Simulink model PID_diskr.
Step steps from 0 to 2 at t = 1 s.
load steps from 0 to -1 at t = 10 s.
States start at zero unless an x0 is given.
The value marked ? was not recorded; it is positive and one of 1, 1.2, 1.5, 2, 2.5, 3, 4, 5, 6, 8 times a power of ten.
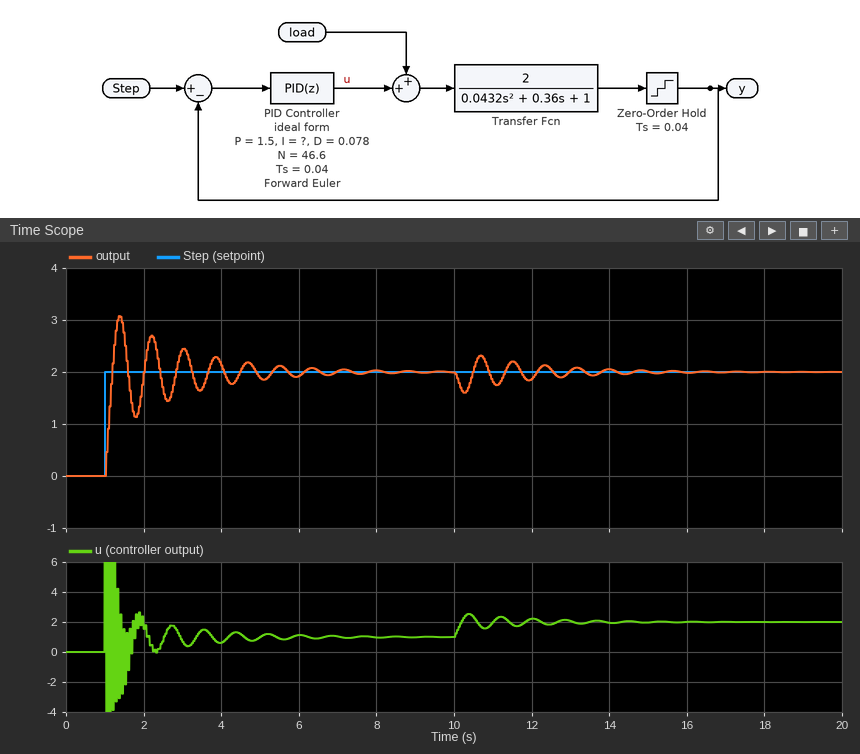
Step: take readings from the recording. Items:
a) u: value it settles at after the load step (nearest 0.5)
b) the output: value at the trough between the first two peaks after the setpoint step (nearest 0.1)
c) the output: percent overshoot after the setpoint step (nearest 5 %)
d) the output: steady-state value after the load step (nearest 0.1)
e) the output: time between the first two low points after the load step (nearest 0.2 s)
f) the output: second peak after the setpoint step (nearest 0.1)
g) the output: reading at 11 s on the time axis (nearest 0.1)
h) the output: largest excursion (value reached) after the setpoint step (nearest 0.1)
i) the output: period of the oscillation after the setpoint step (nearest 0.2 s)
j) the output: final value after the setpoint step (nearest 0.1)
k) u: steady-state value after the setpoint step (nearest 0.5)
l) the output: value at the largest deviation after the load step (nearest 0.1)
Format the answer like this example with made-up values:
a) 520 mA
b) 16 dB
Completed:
a) 2.0
b) 1.1
c) 55 %
d) 2.0
e) 0.8 s
f) 2.7
g) 1.8
h) 3.1
i) 0.8 s
j) 2.0
k) 1.0
l) 1.6
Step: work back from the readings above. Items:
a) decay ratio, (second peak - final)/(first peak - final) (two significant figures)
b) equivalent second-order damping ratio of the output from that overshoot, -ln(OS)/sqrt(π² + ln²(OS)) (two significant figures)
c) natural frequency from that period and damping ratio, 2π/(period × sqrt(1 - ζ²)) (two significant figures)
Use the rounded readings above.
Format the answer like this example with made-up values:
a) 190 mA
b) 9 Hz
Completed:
a) 0.64
b) 0.19
c) 8.0 rad/s
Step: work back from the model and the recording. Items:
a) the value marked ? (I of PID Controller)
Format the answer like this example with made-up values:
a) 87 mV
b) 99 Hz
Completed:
a) 10
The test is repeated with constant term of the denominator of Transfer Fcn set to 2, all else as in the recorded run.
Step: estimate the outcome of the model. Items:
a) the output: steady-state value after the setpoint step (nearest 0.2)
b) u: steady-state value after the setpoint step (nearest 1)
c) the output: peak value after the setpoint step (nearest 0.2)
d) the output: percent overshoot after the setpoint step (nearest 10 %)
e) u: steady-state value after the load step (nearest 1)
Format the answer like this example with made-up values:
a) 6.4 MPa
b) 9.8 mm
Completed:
a) 2.0
b) 2
c) 2.6
d) 30 %
e) 3
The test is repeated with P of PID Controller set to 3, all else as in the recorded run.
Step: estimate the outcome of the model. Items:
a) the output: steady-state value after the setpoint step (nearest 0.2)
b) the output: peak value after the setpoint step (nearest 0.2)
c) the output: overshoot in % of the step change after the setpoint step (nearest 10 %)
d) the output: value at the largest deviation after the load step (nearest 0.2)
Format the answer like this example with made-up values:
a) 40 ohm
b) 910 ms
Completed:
a) 2.0
b) 2.8
c) 40 %
d) 1.8
